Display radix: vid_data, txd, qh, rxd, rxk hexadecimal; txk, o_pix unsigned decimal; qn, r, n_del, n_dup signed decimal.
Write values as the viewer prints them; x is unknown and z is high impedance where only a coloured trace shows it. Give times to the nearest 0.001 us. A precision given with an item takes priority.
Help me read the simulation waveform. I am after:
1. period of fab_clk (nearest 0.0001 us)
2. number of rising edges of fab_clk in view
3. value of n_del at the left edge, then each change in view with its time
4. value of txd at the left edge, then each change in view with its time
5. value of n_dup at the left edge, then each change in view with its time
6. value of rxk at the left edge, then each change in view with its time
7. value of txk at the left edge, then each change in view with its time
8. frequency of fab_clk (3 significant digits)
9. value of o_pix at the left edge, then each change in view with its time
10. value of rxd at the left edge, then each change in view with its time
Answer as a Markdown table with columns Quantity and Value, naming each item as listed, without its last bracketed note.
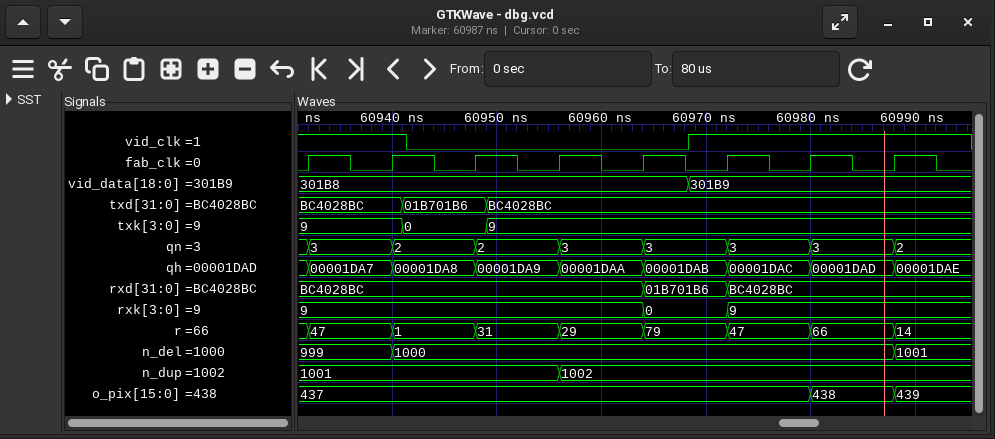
| Quantity | Value |
|---|---|
| period of fab_clk | 0.008 us |
| number of rising edges of fab_clk in view | 8 |
| value of n_del at the left edge, then each change in view with its time | 999, 1000 at 60.94 us, 1001 at 60.988 us |
| value of txd at the left edge, then each change in view with its time | BC4028BC, 01B701B6 at 60.941 us, BC4028BC at 60.949 us |
| value of n_dup at the left edge, then each change in view with its time | 1001, 1002 at 60.956 us |
| value of rxk at the left edge, then each change in view with its time | 9, 0 at 60.964 us, 9 at 60.972 us |
| value of txk at the left edge, then each change in view with its time | 9, 0 at 60.941 us, 9 at 60.949 us |
| frequency of fab_clk | 125 MHz |
| value of o_pix at the left edge, then each change in view with its time | 437, 438 at 60.98 us, 439 at 60.988 us |
| value of rxd at the left edge, then each change in view with its time | BC4028BC, 01B701B6 at 60.964 us, BC4028BC at 60.972 us |
